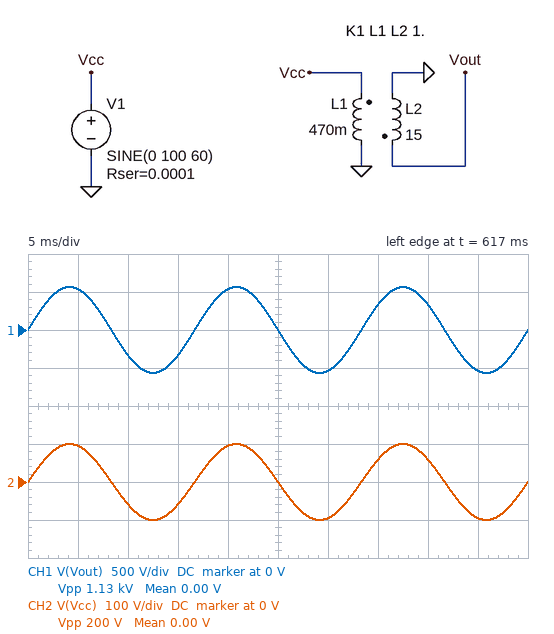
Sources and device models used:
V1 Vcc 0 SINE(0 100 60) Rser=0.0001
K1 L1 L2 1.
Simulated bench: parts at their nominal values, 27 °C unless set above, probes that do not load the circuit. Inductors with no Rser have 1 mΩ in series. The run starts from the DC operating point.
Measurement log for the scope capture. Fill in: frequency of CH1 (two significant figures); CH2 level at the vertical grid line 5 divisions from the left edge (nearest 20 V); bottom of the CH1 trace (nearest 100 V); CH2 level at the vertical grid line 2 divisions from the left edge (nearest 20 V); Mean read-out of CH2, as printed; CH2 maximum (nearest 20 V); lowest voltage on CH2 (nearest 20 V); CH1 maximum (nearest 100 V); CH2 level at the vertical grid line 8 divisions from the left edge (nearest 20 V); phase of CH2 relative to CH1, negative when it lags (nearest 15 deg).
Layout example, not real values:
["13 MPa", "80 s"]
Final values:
["60 Hz", "0 V", "-600 V", "-60 V", "0.00 V", "100 V", "-100 V", "600 V", "60 V", "0 deg"]
